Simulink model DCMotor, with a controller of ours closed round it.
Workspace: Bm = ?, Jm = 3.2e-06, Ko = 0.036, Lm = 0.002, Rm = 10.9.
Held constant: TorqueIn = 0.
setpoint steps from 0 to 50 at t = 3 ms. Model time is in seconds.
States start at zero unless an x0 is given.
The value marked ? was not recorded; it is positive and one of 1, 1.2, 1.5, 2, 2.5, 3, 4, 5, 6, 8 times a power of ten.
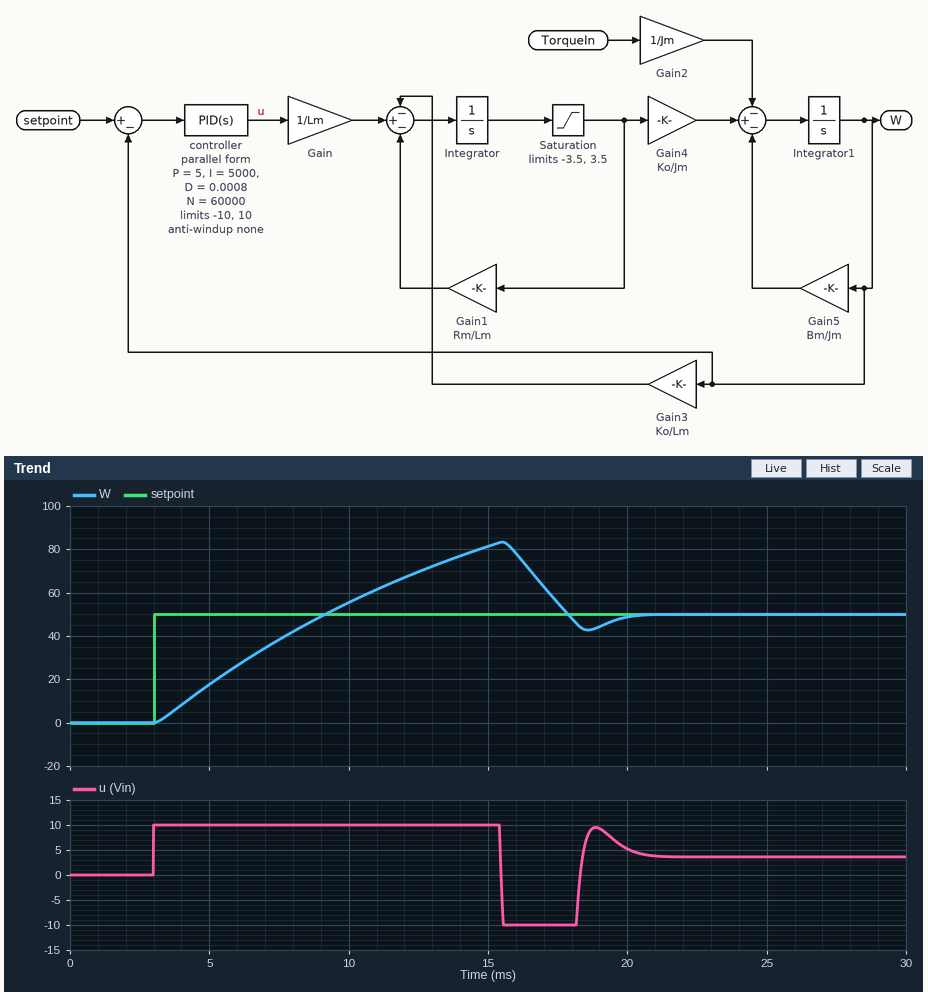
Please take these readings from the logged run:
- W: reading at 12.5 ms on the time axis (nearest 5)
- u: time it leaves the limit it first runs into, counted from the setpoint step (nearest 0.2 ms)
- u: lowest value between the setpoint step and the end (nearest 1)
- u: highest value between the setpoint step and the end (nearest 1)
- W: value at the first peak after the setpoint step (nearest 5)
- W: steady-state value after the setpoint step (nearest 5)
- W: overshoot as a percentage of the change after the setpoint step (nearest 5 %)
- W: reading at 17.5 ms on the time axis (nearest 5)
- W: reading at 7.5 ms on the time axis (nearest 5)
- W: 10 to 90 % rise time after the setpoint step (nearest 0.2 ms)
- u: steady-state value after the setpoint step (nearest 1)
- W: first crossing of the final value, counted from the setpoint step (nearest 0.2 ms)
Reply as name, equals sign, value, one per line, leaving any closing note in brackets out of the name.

W: reading at 12.5 ms on the time axis = 70
u: time it leaves the limit it first runs into, counted from the setpoint step = 12.4 ms
u: lowest value between the setpoint step and the end = -10
u: highest value between the setpoint step and the end = 10
W: value at the first peak after the setpoint step = 85
W: steady-state value after the setpoint step = 50
W: overshoot as a percentage of the change after the setpoint step = 65 %
W: reading at 17.5 ms on the time axis = 55
W: reading at 7.5 ms on the time axis = 40
W: 10 to 90 % rise time after the setpoint step = 4.8 ms
u: steady-state value after the setpoint step = 4
W: first crossing of the final value, counted from the setpoint step = 6.2 ms
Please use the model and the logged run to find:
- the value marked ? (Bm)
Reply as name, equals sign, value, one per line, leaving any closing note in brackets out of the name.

the value marked ? = 0.00012
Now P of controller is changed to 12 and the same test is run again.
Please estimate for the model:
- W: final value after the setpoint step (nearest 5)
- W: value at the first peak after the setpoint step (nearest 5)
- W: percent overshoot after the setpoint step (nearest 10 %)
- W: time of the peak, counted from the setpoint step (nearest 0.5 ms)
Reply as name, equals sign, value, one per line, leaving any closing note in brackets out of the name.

W: final value after the setpoint step = 50
W: value at the first peak after the setpoint step = 80
W: percent overshoot after the setpoint step = 60 %
W: time of the peak, counted from the setpoint step = 11.5 ms
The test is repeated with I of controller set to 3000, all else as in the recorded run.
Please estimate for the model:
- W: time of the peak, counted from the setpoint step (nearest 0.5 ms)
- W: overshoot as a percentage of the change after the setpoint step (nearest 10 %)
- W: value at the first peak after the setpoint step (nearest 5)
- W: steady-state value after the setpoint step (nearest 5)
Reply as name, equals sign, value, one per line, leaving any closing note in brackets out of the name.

W: time of the peak, counted from the setpoint step = 12.0 ms
W: overshoot as a percentage of the change after the setpoint step = 60 %
W: value at the first peak after the setpoint step = 80
W: steady-state value after the setpoint step = 50
